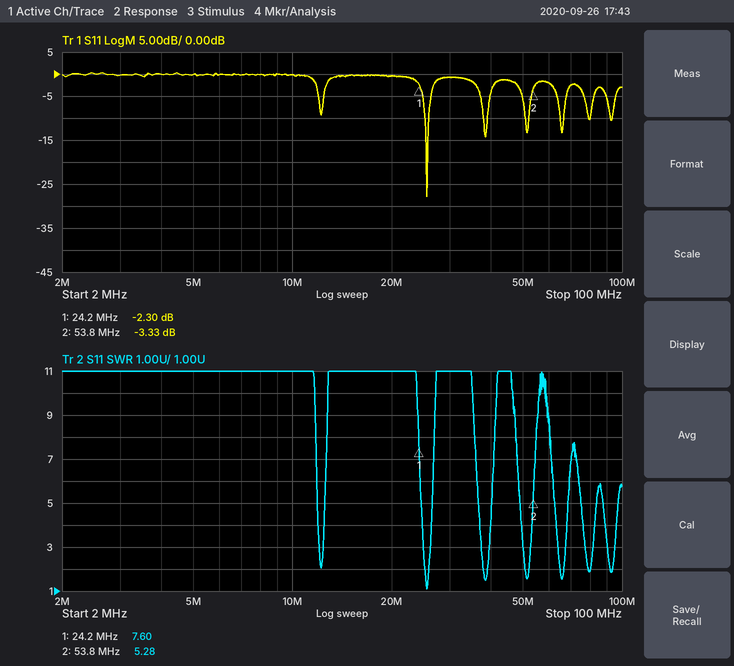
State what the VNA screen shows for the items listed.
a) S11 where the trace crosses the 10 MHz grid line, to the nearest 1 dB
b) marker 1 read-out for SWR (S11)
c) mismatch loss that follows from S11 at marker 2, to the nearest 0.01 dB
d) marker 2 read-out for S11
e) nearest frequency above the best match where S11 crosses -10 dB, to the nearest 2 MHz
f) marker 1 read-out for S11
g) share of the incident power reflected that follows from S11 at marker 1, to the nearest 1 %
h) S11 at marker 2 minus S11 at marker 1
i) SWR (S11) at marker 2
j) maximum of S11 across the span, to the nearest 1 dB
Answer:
0 dB
7.60
2.71 dB
-3.33 dB
26 MHz
-2.30 dB
59 %
-1.03 dB
5.28
0 dB
